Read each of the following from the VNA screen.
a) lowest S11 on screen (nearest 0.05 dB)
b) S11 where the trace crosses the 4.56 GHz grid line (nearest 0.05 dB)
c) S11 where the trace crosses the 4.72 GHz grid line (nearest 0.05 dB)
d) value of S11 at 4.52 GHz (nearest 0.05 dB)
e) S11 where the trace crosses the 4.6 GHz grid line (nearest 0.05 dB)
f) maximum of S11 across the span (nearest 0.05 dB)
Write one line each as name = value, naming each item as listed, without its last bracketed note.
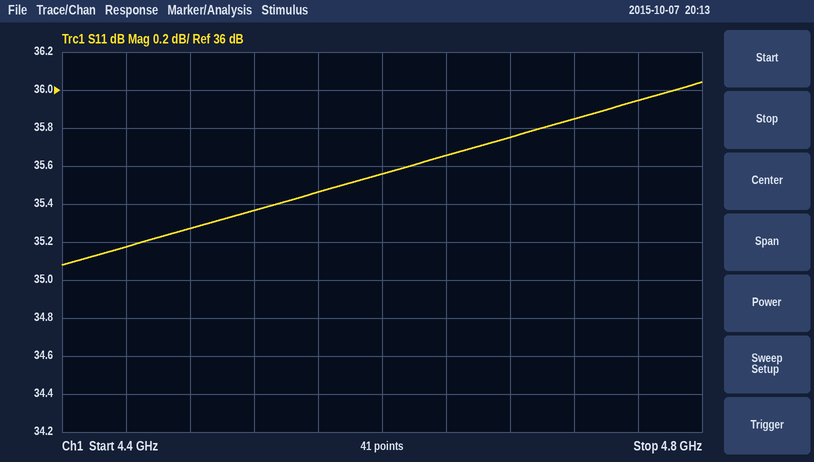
lowest S11 on screen = 35.10 dB
S11 where the trace crosses the 4.56 GHz grid line = 35.45 dB
S11 where the trace crosses the 4.72 GHz grid line = 35.85 dB
value of S11 at 4.52 GHz = 35.35 dB
S11 where the trace crosses the 4.6 GHz grid line = 35.55 dB
maximum of S11 across the span = 36.05 dB
